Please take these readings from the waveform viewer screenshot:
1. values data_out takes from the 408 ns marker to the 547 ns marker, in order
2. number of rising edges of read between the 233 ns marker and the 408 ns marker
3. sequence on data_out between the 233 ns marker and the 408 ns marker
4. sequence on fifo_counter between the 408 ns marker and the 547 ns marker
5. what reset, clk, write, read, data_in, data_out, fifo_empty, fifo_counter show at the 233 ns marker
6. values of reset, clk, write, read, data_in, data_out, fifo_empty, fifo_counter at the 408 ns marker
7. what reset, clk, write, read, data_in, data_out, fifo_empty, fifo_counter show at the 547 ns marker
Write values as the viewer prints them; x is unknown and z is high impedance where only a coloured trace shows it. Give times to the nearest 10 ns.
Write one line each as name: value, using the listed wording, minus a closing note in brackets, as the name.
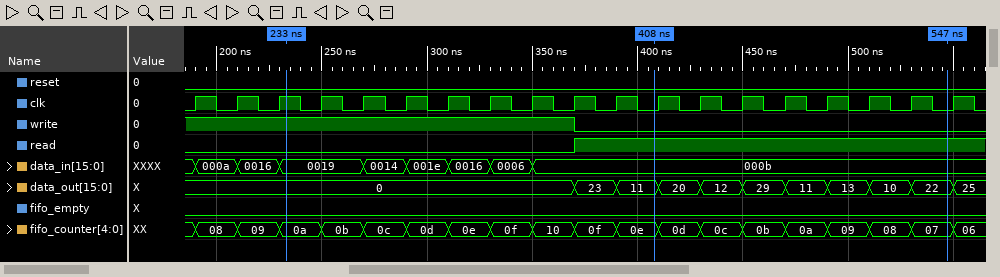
values data_out takes from the 408 ns marker to the 547 ns marker, in order: 11, 20, 12, 29, 11, 13, 10, 22
number of rising edges of read between the 233 ns marker and the 408 ns marker: 1
sequence on data_out between the 233 ns marker and the 408 ns marker: 0, 23, 11
sequence on fifo_counter between the 408 ns marker and the 547 ns marker: 0e, 0d, 0c, 0b, 0a, 09, 08, 07
what reset, clk, write, read, data_in, data_out, fifo_empty, fifo_counter show at the 233 ns marker: reset=0, clk=1, write=1, read=0, data_in=0019, data_out=0, fifo_empty=0, fifo_counter=0a
values of reset, clk, write, read, data_in, data_out, fifo_empty, fifo_counter at the 408 ns marker: reset=0, clk=0, write=0, read=1, data_in=000b, data_out=11, fifo_empty=0, fifo_counter=0e
what reset, clk, write, read, data_in, data_out, fifo_empty, fifo_counter show at the 547 ns marker: reset=0, clk=0, write=0, read=1, data_in=000b, data_out=22, fifo_empty=0, fifo_counter=07
